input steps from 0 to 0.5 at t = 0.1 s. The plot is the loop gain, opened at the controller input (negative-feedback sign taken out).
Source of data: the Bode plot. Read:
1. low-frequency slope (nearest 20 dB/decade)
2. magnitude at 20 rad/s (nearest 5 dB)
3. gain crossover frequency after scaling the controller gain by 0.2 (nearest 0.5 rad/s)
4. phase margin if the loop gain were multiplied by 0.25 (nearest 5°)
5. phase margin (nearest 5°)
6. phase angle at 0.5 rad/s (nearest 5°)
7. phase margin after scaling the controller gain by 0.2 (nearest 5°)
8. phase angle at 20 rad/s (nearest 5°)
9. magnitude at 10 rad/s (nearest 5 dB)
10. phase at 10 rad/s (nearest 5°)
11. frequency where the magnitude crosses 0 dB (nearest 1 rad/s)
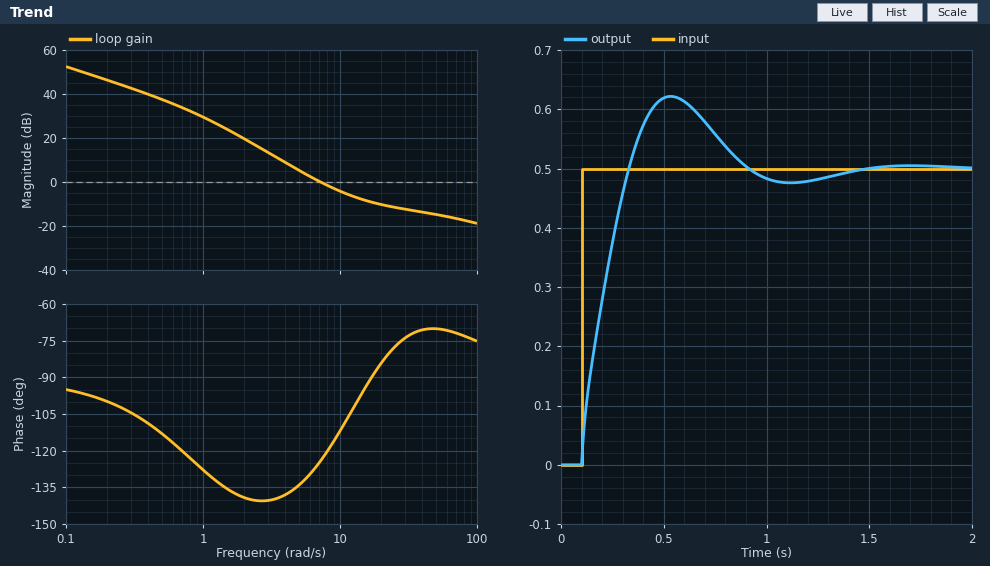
-20 dB/decade
-10 dB
3.0 rad/s
40°
55°
-115°
40°
-85°
-5 dB
-110°
7 rad/s
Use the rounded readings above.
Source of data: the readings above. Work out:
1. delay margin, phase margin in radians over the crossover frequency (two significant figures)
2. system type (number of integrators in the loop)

0.14 s
1
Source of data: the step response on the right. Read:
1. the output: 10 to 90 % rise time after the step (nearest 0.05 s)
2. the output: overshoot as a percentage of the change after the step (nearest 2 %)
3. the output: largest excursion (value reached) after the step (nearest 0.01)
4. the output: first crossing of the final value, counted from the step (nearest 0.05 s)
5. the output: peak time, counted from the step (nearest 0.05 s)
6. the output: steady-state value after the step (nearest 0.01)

0.20 s
24 %
0.62
0.25 s
0.45 s
0.50
